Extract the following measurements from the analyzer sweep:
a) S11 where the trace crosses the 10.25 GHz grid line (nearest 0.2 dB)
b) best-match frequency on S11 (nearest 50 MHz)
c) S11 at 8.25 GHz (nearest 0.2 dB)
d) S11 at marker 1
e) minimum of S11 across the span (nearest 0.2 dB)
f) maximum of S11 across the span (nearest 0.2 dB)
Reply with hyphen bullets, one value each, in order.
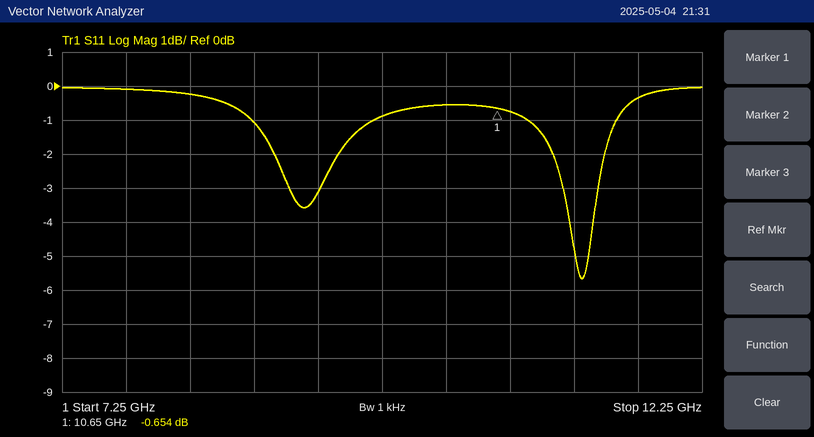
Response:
- -0.6 dB
- 11.30 GHz
- -0.2 dB
- -0.654 dB
- -5.6 dB
- 0.0 dB
